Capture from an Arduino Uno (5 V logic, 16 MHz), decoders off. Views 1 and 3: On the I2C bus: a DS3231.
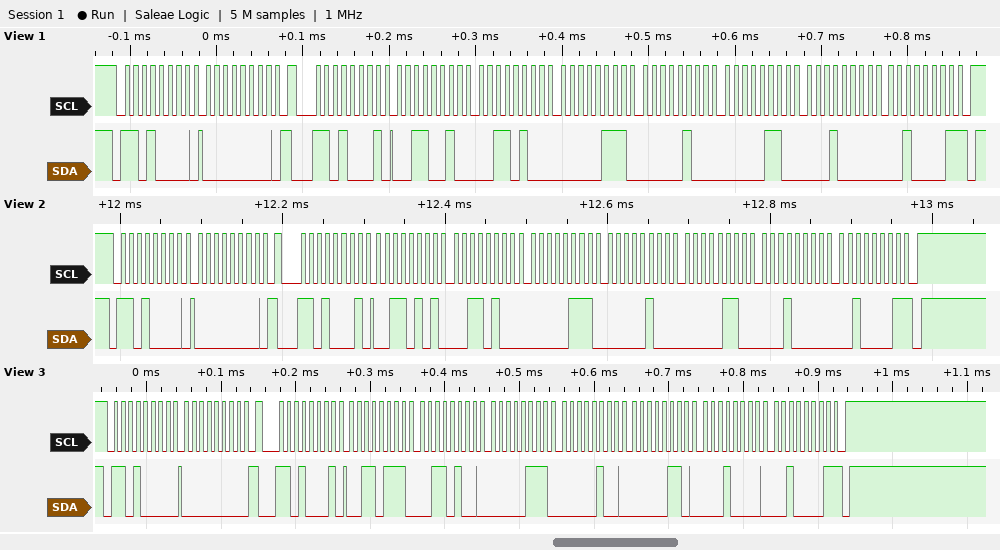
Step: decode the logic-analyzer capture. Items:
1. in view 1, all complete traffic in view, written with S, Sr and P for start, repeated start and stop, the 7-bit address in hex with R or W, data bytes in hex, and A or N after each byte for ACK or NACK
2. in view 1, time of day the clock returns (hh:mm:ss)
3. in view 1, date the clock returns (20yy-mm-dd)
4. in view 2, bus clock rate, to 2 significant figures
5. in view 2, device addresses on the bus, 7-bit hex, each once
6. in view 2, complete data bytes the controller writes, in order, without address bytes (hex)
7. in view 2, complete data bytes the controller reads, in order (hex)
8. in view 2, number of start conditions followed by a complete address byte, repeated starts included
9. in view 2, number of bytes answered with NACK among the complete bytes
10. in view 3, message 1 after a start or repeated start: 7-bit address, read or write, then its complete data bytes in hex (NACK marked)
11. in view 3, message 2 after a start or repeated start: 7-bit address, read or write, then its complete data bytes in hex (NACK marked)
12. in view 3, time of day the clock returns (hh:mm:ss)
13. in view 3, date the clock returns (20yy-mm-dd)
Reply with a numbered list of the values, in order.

1. S 68W A 00 A Sr 68R A 32 A 34 A 07 A 04 A 06 A 10 A 21 N P
2. 07:34:32
3. 2021-10-06
4. 100 kHz
5. 0x68
6. 00
7. 35 34 07 04 06 10 21
8. 2
9. 1
10. 0x68 write: 00
11. 0x68 read: 37 34 07 04 06 10 21 NACK
12. 07:34:37
13. 2021-10-06
